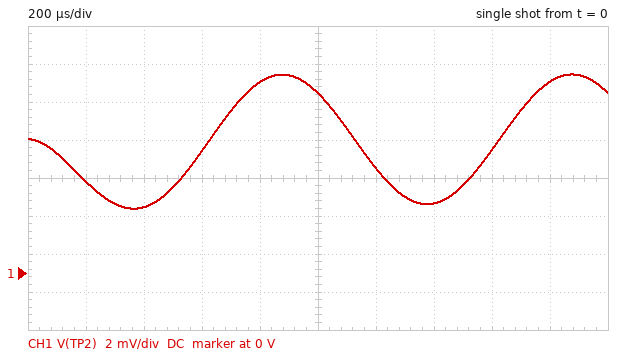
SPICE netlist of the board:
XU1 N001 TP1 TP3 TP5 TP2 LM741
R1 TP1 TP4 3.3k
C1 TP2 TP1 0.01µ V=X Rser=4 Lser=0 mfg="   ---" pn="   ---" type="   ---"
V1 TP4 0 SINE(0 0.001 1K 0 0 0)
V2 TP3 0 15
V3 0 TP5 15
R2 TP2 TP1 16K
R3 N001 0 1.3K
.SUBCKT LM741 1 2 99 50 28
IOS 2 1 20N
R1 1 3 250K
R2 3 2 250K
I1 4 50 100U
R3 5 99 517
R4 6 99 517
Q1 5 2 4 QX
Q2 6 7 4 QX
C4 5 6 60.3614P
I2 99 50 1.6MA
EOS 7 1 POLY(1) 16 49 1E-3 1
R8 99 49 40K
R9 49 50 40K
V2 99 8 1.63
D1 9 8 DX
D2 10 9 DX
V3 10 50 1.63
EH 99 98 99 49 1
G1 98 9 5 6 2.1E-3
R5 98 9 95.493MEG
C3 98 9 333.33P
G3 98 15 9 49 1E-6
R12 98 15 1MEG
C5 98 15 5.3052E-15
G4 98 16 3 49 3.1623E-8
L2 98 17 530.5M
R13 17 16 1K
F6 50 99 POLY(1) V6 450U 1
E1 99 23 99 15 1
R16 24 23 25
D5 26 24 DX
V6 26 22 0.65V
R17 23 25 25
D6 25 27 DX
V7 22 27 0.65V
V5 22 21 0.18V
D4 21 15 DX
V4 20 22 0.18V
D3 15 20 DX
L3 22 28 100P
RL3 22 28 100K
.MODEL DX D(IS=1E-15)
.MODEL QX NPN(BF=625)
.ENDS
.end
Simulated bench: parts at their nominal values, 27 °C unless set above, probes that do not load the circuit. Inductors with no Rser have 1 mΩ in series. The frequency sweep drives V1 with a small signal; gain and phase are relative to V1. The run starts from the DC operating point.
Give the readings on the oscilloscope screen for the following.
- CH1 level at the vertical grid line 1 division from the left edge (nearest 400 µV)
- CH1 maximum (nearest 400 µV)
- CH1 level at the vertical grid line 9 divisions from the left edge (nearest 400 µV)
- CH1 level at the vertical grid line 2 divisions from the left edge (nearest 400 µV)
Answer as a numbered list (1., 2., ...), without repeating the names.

1. 4.8 mV
2. 10.4 mV
3. 10.0 mV
4. 3.6 mV
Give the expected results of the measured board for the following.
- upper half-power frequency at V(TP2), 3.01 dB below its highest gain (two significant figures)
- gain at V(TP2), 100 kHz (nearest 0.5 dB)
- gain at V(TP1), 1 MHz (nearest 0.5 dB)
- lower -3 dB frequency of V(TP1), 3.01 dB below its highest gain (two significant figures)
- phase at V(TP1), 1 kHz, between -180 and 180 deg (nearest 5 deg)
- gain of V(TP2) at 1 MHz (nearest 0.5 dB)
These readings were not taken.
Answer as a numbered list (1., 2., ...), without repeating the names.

1. 990 Hz
2. -25.5 dB
3. -25.5 dB
4. 900 kHz
5. 45 deg
6. -25.0 dB
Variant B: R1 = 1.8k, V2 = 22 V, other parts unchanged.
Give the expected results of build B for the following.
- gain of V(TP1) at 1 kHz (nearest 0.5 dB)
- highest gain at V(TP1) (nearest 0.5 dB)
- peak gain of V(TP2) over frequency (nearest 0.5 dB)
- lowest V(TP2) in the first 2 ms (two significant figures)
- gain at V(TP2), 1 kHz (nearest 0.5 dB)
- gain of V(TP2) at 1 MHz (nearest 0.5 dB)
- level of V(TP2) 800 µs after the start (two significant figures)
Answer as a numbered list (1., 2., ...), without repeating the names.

1. -44.0 dB
2. -18.5 dB
3. 19.0 dB
4. 3.2 mV
5. 16.0 dB
6. -20.0 dB
7. 15 mV
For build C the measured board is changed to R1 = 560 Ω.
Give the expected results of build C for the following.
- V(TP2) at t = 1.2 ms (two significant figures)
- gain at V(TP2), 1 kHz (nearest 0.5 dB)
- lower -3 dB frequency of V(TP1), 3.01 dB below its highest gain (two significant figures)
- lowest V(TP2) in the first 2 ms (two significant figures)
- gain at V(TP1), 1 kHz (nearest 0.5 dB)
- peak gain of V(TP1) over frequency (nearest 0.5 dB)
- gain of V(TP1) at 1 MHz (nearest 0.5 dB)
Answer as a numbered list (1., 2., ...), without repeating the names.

1. 20 mV
2. 26.0 dB
3. 750 kHz
4. 7.6 mV
5. -34.0 dB
6. -10.0 dB
7. -11.5 dB
